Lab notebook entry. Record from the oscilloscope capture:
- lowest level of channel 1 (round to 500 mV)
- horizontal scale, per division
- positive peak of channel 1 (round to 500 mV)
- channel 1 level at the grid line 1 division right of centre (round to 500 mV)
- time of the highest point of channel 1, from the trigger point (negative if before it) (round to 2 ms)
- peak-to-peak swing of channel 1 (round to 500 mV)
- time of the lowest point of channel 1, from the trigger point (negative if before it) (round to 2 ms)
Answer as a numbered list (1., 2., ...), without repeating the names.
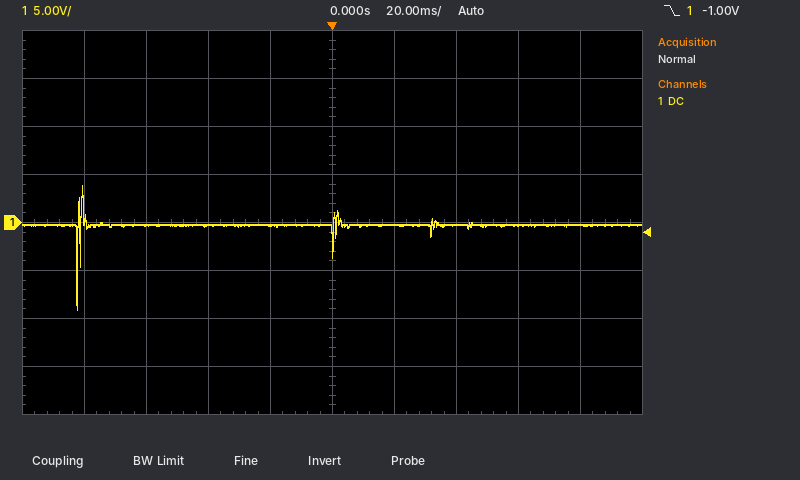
1. -9.0 V
2. 20 ms
3. 4.0 V
4. 0.0 V
5. -80 ms
6. 13.0 V
7. -82 ms
